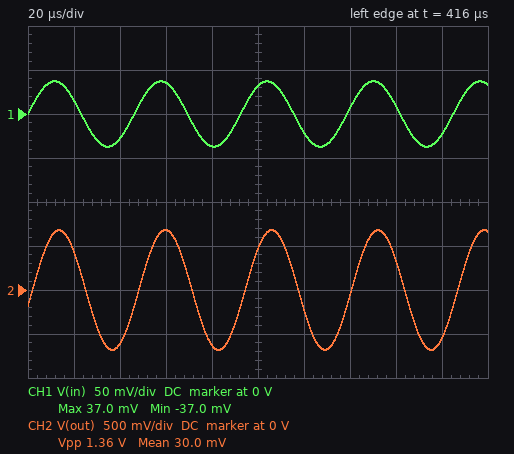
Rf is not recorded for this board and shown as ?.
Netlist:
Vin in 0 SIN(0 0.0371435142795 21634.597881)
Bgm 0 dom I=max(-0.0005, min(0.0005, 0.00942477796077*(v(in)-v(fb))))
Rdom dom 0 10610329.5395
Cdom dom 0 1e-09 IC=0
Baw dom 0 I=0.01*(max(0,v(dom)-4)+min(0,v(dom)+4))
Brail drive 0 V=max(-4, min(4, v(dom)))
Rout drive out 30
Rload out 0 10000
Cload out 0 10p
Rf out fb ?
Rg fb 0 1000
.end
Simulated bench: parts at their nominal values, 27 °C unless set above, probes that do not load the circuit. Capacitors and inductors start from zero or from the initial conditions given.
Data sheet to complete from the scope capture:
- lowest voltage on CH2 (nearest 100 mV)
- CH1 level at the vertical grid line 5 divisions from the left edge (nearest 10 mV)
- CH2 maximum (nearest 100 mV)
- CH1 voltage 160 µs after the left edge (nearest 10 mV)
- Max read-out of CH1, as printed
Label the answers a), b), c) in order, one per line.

a) -700 mV
b) 30 mV
c) 700 mV
d) 10 mV
e) 37.0 mV
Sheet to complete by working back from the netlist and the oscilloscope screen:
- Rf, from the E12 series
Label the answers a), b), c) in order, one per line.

a) 18 kΩ
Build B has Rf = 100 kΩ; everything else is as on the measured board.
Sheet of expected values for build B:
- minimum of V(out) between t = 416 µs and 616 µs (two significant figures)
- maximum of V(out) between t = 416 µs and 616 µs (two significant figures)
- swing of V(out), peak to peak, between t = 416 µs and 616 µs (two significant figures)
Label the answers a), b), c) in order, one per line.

a) -2.1 V
b) 2.1 V
c) 4.2 V
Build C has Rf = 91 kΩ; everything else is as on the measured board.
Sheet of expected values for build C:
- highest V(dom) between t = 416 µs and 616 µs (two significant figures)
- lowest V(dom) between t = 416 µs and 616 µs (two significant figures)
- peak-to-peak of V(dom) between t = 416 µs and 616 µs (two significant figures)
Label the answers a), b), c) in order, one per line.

a) 2.1 V
b) -2.1 V
c) 4.1 V
